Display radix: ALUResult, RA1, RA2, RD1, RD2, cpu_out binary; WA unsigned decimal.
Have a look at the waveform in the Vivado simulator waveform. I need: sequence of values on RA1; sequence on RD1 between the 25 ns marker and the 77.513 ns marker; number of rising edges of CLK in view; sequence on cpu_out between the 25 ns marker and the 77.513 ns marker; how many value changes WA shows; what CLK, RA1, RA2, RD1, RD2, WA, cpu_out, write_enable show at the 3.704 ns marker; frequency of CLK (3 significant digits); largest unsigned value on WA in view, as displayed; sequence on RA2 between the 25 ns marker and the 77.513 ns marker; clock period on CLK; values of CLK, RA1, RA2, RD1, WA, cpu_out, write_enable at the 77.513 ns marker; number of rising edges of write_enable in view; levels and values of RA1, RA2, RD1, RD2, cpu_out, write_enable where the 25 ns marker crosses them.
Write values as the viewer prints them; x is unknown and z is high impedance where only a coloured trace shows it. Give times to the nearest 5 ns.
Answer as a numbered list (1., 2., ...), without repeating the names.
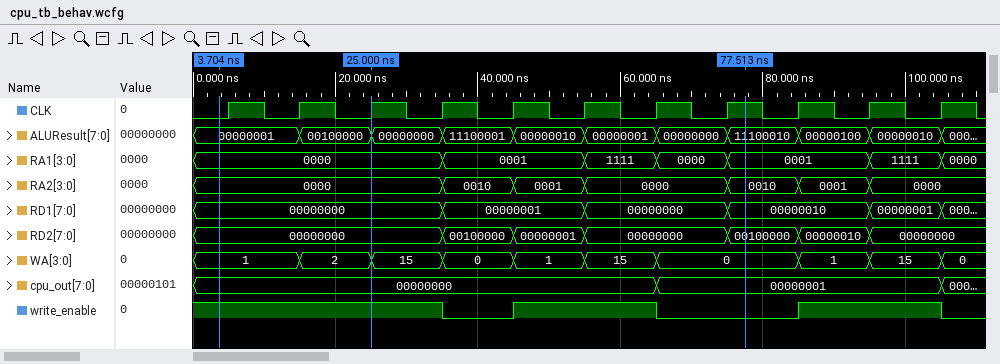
1. 0000, 0001, 1111, 0000, 0001, 1111, 0000
2. 00000000, 00000001, 00000000, 00000010
3. 11
4. 00000000, 00000001
5. 9
6. CLK=0, RA1=0000, RA2=0000, RD1=00000000, RD2=00000000, WA=1, cpu_out=00000000, write_enable=1
7. 100 MHz
8. 15
9. 0000, 0010, 0001, 0000, 0010
10. 10 ns
11. CLK=1, RA1=0001, RA2=0010, RD1=00000010, WA=0, cpu_out=00000001, write_enable=0
12. 2
13. RA1=0000, RA2=0000, RD1=00000000, RD2=00000000, cpu_out=00000000, write_enable=1
